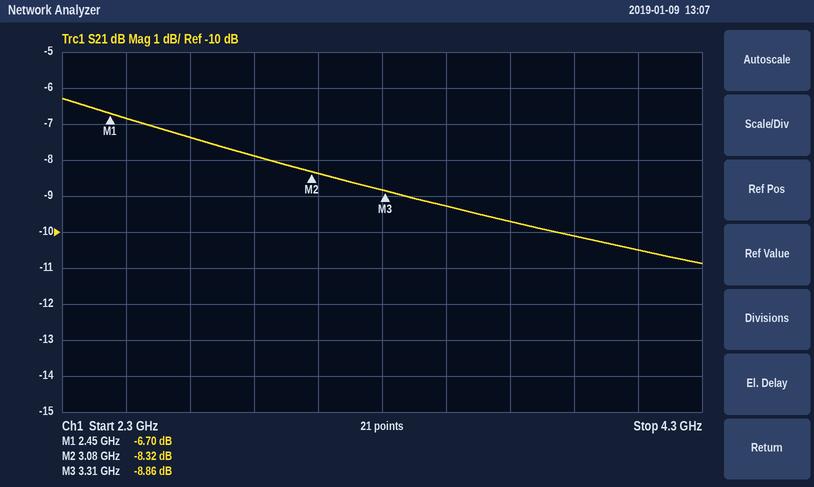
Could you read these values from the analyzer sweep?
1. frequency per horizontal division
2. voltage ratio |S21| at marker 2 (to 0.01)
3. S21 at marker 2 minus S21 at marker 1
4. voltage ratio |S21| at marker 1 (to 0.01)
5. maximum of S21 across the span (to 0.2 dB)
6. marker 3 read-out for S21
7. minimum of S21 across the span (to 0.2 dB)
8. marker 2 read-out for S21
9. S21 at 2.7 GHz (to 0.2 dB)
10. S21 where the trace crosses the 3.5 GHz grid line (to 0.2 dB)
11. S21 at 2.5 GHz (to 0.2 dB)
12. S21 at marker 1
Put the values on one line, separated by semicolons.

200 MHz; 0.38; -1.62 dB; 0.46; -6.2 dB; -8.86 dB; -10.8 dB; -8.32 dB; -7.4 dB; -9.2 dB; -6.8 dB; -6.70 dB
